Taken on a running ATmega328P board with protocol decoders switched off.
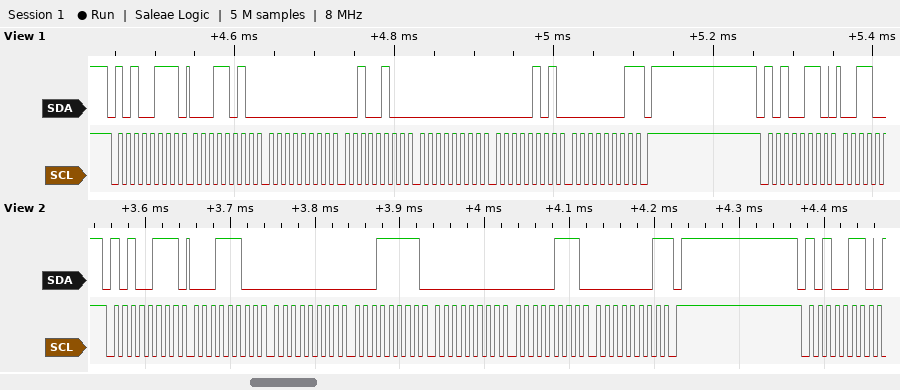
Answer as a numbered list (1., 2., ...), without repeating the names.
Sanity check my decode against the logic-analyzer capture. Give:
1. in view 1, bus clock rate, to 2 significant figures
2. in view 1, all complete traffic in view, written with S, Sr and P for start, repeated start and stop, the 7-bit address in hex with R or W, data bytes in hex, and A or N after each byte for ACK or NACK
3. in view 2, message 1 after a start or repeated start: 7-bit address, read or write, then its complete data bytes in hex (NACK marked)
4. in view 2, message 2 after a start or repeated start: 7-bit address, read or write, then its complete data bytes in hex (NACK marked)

1. 100 kHz
2. S 53R A 1A A 00 A 24 A 00 A 05 A 01 N P S 53W A
3. 0x53 read: 1C 00 1F 00 07 01 NACK
4. 0x53 write
